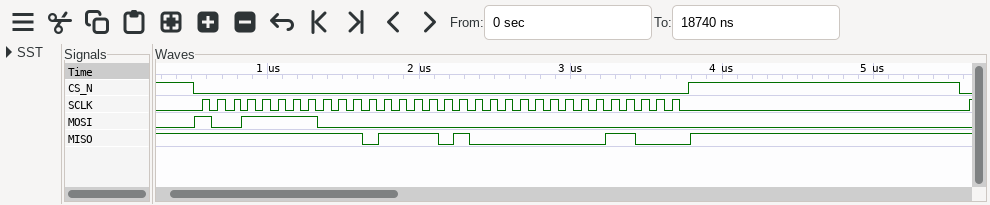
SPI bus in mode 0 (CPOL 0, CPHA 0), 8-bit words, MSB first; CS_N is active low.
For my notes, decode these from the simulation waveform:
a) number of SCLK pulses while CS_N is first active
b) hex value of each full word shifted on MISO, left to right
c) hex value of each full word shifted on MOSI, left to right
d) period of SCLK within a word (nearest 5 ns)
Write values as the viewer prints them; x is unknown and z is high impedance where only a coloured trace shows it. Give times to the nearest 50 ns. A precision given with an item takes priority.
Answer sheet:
32
FF, EF, 40, 18
9F, 00, 00, 00
100 ns
